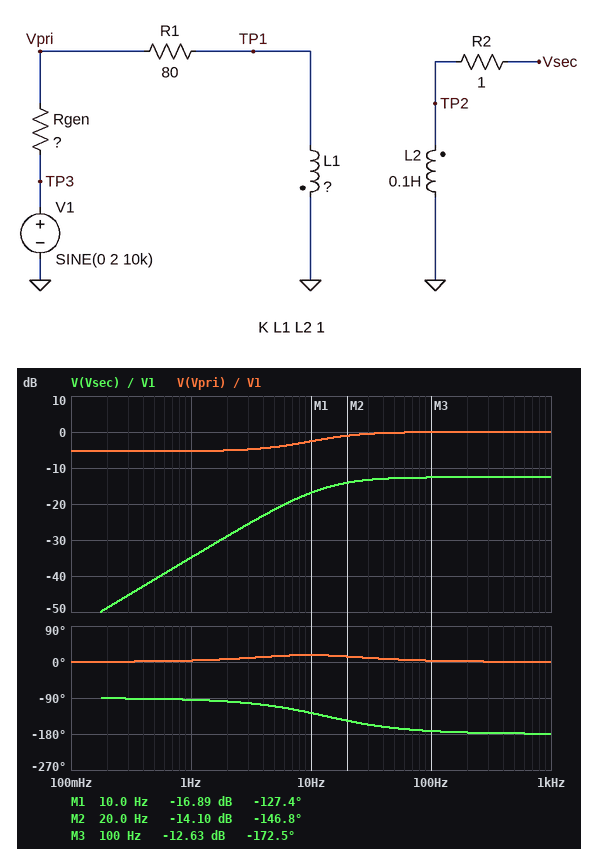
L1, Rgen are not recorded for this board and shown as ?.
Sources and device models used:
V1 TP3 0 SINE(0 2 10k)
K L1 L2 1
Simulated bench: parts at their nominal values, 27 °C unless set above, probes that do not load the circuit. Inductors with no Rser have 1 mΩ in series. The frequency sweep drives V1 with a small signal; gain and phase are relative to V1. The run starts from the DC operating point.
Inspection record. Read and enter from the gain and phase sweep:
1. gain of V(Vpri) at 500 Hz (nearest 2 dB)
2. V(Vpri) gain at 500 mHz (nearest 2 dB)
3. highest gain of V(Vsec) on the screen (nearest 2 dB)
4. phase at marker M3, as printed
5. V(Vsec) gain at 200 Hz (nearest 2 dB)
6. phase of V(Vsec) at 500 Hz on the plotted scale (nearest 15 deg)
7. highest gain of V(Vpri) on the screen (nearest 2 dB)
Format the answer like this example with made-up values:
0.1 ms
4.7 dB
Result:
0 dB
-6 dB
-12 dB
-172.5 deg
-12 dB
-180 deg
0 dB
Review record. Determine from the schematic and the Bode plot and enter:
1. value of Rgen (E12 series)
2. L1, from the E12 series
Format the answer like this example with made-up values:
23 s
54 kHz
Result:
68 Ω
1.8 H
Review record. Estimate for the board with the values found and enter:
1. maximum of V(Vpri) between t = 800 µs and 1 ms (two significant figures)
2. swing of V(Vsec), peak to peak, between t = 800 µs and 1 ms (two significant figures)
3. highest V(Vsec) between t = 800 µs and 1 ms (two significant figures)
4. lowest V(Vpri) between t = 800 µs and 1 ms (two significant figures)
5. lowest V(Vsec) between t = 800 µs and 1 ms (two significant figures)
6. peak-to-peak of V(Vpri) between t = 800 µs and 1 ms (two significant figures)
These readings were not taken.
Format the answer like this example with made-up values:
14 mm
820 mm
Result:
2.0 V
940 mV
470 mV
-2.0 V
-470 mV
4.0 V
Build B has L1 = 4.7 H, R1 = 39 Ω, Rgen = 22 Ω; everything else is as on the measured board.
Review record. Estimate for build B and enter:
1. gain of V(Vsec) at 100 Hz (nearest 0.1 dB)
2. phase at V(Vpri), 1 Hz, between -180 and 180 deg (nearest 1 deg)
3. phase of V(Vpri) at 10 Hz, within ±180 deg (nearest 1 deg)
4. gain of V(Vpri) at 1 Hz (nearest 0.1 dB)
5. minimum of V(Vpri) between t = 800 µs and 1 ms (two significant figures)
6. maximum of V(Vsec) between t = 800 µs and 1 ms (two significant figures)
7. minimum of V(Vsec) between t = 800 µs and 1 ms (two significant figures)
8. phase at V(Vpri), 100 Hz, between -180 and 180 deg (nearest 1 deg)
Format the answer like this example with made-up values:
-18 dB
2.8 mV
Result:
-16.7 dB
11 deg
4 deg
-2.8 dB
-2.0 V
290 mV
-290 mV
0 deg
